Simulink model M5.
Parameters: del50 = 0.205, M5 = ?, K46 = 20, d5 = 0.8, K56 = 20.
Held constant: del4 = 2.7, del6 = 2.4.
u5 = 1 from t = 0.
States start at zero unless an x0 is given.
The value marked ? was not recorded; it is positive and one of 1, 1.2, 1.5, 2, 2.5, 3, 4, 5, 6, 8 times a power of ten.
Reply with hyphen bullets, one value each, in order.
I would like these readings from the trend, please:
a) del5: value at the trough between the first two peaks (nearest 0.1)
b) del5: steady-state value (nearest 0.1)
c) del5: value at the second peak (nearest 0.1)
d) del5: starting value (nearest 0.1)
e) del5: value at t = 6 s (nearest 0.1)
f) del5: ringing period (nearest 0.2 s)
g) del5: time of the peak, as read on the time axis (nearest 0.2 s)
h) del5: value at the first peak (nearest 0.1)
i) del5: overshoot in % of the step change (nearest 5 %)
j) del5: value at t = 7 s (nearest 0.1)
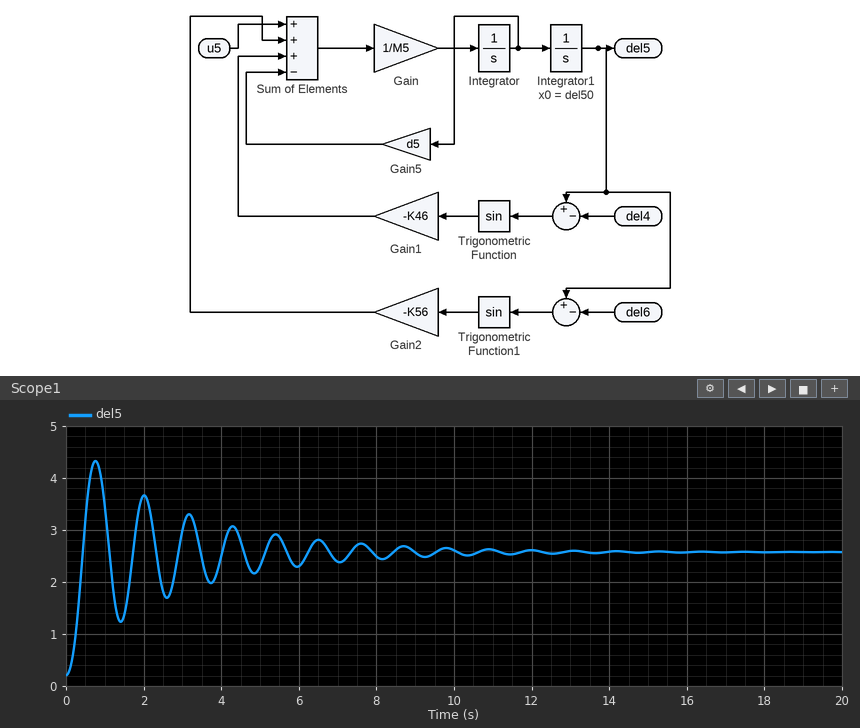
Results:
- 1.2
- 2.6
- 3.7
- 0.2
- 2.3
- 1.2 s
- 0.8 s
- 4.3
- 75 %
- 2.4
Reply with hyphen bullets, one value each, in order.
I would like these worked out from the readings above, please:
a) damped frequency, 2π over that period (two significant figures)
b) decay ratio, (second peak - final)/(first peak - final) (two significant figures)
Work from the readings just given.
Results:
- 5.2 rad/s
- 0.65
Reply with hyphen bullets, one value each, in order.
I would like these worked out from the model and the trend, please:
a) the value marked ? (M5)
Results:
- 1.2
